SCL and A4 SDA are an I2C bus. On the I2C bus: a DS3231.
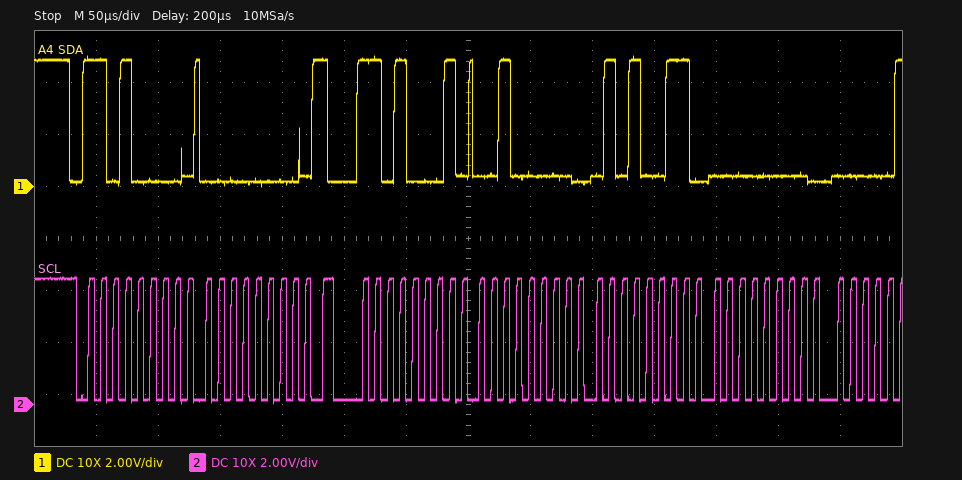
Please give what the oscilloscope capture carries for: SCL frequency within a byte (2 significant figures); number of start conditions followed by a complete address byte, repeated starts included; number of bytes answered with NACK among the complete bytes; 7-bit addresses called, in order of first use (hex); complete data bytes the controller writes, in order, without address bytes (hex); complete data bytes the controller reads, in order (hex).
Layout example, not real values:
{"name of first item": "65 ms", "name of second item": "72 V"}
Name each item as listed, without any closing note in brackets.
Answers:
{"SCL frequency within a byte": "100 kHz", "number of start conditions followed by a complete address byte, repeated starts included": "2", "number of bytes answered with NACK among the complete bytes": "0", "7-bit addresses called, in order of first use": "0x68", "complete data bytes the controller writes, in order, without address bytes": "00", "complete data bytes the controller reads, in order": "20 53 00"}
